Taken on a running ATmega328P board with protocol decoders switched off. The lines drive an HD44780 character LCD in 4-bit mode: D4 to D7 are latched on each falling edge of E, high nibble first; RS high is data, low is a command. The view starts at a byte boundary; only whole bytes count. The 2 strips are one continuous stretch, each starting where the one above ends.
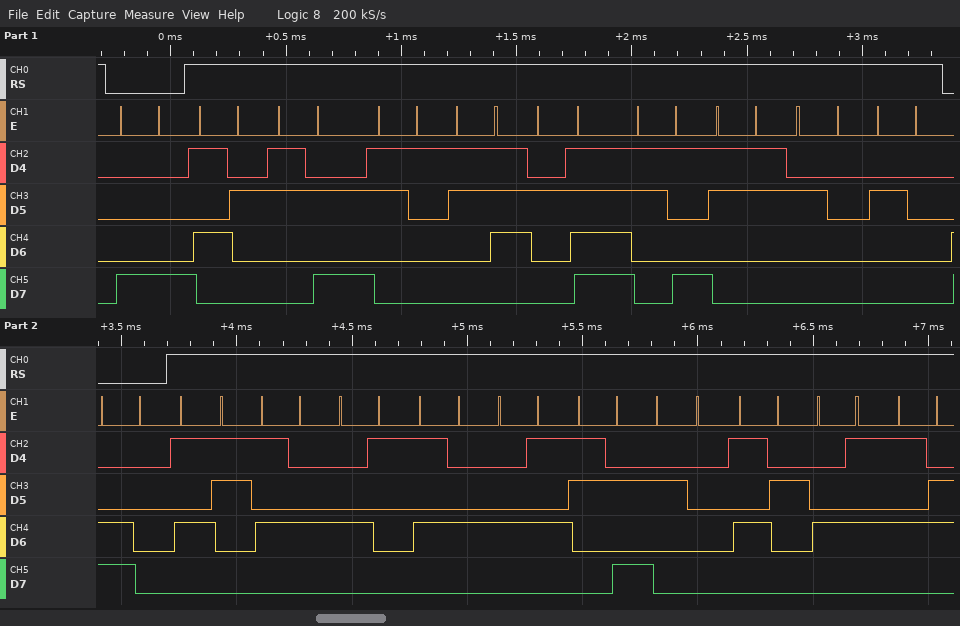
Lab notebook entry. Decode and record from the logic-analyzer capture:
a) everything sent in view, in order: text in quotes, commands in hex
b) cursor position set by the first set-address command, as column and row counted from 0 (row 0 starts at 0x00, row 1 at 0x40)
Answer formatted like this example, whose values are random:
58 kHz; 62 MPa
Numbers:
0x88 "R:17/93  " 0xC0 "STATE: REV"; column 8, row 0
